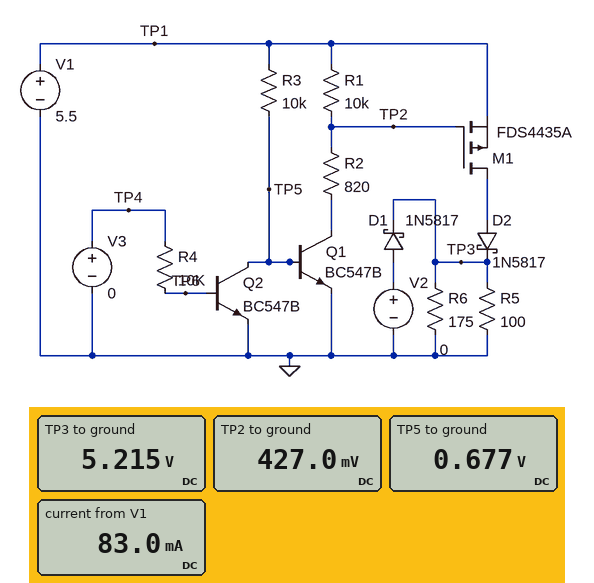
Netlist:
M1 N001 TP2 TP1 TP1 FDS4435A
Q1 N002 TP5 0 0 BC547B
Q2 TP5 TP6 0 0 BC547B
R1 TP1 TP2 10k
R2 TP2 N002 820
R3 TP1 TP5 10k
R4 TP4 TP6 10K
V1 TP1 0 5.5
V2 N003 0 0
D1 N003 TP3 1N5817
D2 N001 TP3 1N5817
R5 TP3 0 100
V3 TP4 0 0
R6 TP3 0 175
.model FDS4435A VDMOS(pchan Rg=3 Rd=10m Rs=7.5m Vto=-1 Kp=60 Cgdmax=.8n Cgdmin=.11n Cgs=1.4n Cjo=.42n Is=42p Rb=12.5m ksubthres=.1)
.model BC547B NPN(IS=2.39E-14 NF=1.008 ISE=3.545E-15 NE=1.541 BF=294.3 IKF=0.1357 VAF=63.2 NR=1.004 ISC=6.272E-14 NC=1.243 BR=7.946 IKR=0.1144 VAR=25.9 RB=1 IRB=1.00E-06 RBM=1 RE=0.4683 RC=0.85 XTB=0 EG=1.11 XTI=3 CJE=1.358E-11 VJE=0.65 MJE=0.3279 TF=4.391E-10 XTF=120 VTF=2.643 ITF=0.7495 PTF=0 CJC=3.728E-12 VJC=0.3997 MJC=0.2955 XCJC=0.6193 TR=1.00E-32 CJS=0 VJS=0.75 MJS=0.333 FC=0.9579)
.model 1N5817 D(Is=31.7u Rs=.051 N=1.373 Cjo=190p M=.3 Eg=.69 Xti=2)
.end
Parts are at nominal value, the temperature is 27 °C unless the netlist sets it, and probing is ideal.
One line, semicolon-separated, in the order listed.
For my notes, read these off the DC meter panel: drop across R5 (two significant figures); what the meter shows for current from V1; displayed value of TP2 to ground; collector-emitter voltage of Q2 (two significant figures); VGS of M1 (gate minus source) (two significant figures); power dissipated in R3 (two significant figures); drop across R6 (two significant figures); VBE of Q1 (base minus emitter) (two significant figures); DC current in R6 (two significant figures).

5.2 V; 83.0 mA; 427.0 mV; 680 mV; -5.1 V; 2.3 mW; 5.2 V; 680 mV; 30 mA
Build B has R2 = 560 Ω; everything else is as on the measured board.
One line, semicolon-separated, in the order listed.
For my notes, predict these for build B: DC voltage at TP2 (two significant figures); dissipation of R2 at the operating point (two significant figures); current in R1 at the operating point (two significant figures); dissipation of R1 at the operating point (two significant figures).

300 mV; 150 µW; 520 µA; 2.7 mW
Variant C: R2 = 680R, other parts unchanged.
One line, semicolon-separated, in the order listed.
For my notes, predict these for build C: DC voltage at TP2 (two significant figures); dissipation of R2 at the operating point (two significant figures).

360 mV; 180 µW
